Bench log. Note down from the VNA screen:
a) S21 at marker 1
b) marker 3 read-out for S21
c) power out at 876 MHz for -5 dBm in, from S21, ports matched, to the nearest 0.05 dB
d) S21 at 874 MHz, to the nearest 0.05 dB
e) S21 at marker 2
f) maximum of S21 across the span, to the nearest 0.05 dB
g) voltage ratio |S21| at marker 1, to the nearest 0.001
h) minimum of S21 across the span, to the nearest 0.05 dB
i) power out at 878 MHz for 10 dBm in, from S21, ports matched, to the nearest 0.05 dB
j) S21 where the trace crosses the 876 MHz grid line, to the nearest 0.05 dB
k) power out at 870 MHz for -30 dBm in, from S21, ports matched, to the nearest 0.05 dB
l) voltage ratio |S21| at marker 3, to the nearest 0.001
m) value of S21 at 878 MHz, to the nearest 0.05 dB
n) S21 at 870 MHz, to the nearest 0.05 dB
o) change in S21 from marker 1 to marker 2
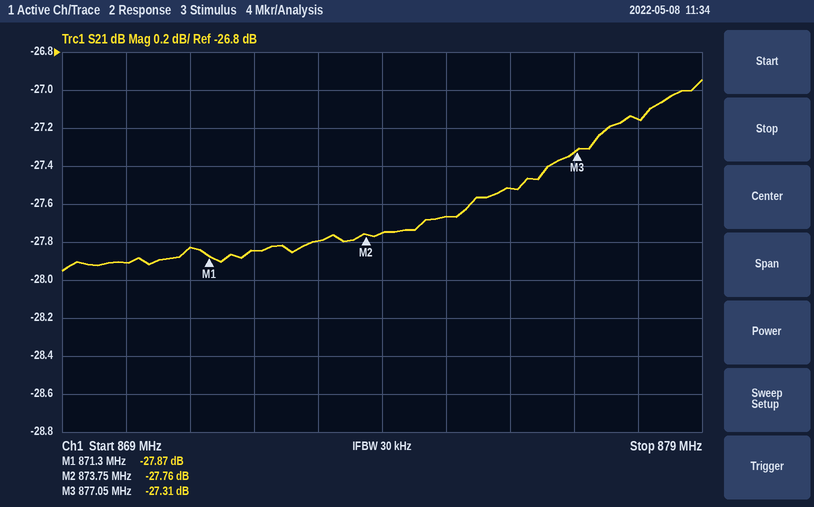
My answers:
-27.87 dB
-27.31 dB
-32.50 dBm
-27.75 dB
-27.76 dB
-26.95 dB
0.040
-27.95 dB
-17.15 dBm
-27.50 dB
-57.90 dBm
0.043
-27.15 dB
-27.90 dB
0.11 dB
